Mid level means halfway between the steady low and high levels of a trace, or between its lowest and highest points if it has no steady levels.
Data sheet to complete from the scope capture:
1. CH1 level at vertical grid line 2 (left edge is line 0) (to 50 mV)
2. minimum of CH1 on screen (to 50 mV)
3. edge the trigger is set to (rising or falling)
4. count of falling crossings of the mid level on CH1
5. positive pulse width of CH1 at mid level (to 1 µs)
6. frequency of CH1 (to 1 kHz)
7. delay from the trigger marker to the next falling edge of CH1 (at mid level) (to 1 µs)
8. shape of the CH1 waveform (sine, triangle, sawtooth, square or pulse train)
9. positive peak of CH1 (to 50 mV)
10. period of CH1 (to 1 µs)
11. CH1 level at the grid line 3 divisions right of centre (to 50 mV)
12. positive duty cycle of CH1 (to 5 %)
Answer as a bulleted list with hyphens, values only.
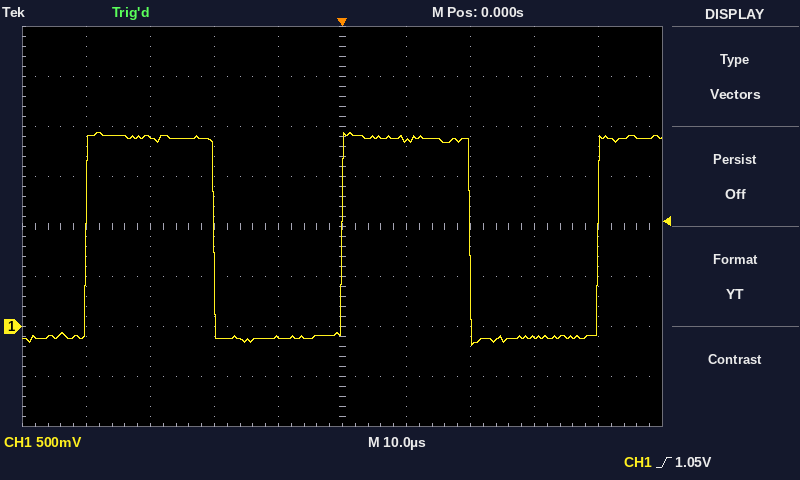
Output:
- 1.90 V
- -200 mV
- rising
- 2
- 20 µs
- 25 kHz
- 20 µs
- square
- 1.95 V
- 40 µs
- -100 mV
- 50 %
